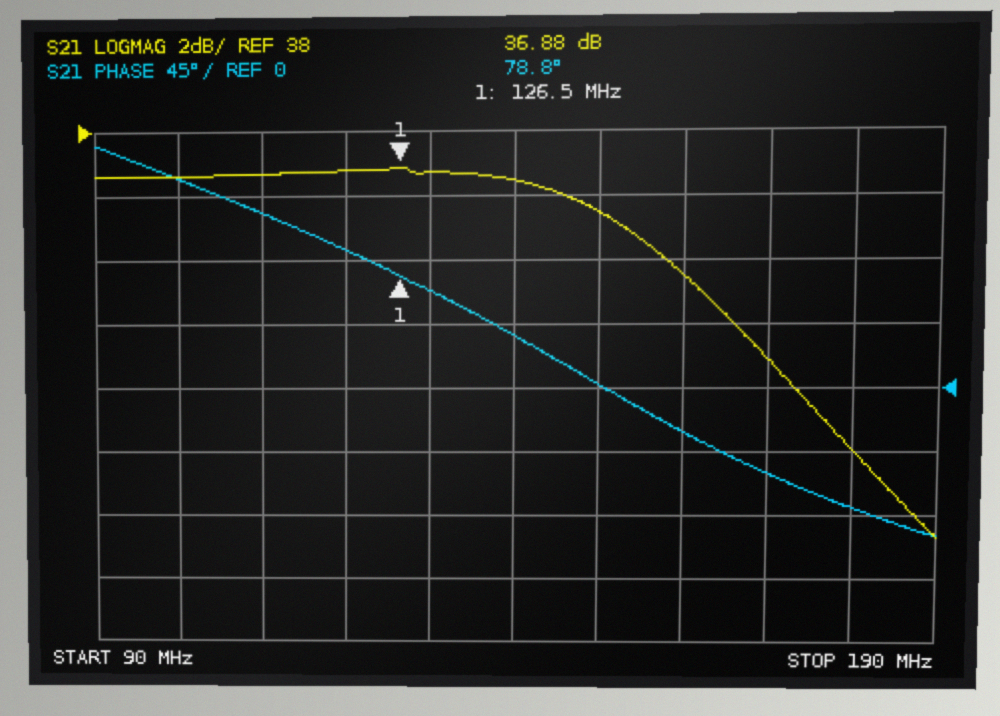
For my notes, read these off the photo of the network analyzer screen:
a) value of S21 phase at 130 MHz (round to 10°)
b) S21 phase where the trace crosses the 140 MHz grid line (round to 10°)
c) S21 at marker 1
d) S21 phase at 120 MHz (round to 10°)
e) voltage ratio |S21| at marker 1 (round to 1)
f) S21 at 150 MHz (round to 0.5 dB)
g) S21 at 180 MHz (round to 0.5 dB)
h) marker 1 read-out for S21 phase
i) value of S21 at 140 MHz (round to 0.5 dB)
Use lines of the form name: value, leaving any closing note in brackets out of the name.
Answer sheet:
value of S21 phase at 130 MHz: 70°
S21 phase where the trace crosses the 140 MHz grid line: 40°
S21 at marker 1: 36.88 dB
S21 phase at 120 MHz: 100°
voltage ratio |S21| at marker 1: 70
S21 at 150 MHz: 35.5 dB
S21 at 180 MHz: 28.0 dB
marker 1 read-out for S21 phase: 78.8°
value of S21 at 140 MHz: 36.5 dB
